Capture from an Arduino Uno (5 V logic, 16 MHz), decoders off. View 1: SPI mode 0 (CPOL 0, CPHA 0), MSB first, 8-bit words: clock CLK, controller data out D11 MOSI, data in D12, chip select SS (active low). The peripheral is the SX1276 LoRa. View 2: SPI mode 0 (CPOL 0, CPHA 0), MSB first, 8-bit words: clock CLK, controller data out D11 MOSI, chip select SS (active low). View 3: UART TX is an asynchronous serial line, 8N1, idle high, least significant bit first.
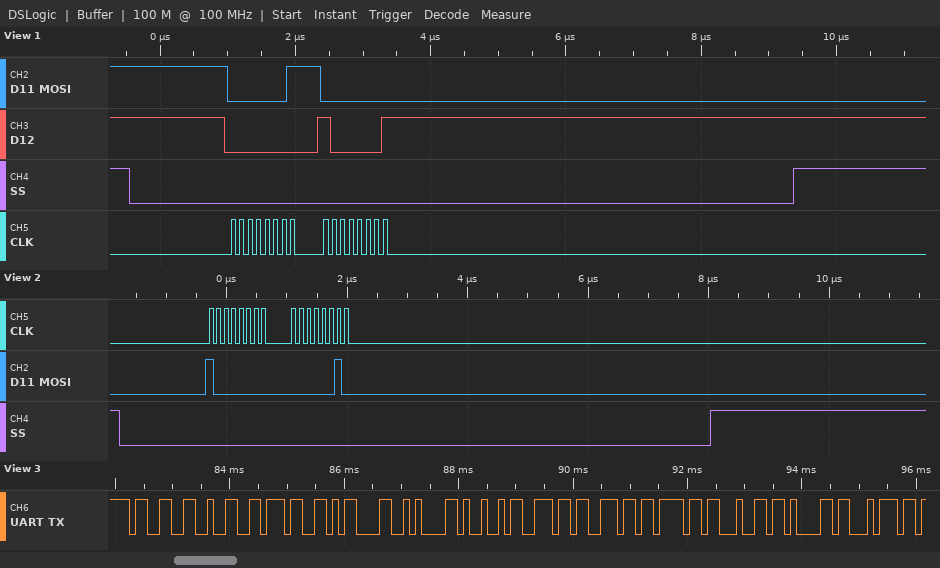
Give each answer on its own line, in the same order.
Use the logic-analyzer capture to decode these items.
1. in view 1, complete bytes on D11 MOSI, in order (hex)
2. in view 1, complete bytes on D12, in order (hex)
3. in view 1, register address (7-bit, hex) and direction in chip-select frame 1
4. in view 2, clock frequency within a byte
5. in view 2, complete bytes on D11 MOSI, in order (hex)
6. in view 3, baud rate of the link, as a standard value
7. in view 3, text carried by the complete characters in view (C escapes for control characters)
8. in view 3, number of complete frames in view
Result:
0x01 0x00
0x00 0x81
0x01 read
8 MHz
80 02
9600 baud
"327\r\nInnodat"
12
